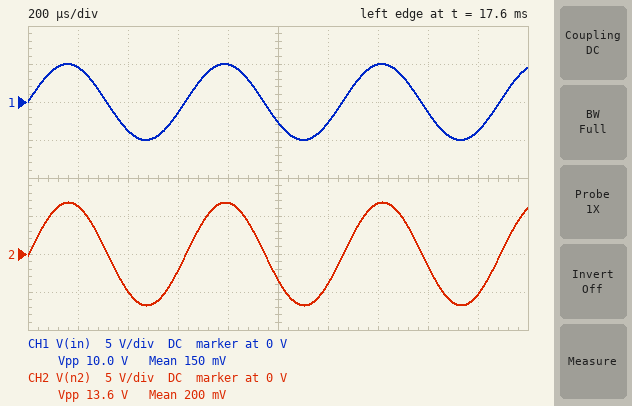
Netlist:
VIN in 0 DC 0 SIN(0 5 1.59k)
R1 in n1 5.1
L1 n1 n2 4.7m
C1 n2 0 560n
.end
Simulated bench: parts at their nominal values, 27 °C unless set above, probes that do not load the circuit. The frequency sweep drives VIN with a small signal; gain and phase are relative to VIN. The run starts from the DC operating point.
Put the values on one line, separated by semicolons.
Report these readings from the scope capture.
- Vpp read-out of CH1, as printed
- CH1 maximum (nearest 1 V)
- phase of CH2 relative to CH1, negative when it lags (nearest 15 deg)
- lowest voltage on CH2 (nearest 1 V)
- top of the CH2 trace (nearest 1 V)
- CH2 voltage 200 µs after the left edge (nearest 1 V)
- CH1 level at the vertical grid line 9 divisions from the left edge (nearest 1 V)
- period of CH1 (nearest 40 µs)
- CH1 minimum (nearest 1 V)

10.0 V; 5 V; 0 deg; -7 V; 7 V; 6 V; -4 V; 640 µs; -5 V
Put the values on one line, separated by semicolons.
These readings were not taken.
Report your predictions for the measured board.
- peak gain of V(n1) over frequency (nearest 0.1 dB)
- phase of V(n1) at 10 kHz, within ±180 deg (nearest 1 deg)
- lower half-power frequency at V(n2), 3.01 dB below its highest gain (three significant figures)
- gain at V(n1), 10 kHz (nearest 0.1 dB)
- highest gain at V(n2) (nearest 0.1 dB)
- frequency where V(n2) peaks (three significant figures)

0 dB; 1 deg; 3.01 kHz; 0 dB; 25.1 dB; 3.10 kHz
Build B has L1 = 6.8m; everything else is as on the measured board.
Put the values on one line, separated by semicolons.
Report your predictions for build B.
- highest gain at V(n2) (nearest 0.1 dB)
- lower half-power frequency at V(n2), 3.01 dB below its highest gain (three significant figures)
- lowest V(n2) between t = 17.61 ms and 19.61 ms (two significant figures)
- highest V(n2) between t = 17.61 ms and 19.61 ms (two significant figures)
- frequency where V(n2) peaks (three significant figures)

26.7 dB; 2.52 kHz; -8.1 V; 8.1 V; 2.58 kHz
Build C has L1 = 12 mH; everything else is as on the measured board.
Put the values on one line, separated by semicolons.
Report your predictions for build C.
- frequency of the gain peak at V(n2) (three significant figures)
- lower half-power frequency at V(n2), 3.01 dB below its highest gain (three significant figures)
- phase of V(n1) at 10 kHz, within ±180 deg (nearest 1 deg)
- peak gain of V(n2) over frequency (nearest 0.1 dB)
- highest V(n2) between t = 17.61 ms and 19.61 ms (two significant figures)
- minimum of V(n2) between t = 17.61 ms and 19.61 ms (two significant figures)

1.94 kHz; 1.91 kHz; 0 deg; 29.2 dB; 15 V; -15 V
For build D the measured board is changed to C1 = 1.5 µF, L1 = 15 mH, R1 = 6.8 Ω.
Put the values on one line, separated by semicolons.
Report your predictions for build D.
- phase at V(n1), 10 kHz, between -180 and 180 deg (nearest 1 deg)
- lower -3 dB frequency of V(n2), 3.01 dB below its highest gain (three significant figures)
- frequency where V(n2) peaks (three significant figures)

0 deg; 1.02 kHz; 1.06 kHz
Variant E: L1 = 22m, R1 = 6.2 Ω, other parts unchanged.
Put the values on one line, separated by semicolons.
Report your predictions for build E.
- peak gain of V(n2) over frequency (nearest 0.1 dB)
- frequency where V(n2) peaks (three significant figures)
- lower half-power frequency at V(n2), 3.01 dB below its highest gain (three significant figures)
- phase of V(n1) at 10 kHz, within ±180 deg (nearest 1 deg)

30.1 dB; 1.43 kHz; 1.41 kHz; 0 deg
